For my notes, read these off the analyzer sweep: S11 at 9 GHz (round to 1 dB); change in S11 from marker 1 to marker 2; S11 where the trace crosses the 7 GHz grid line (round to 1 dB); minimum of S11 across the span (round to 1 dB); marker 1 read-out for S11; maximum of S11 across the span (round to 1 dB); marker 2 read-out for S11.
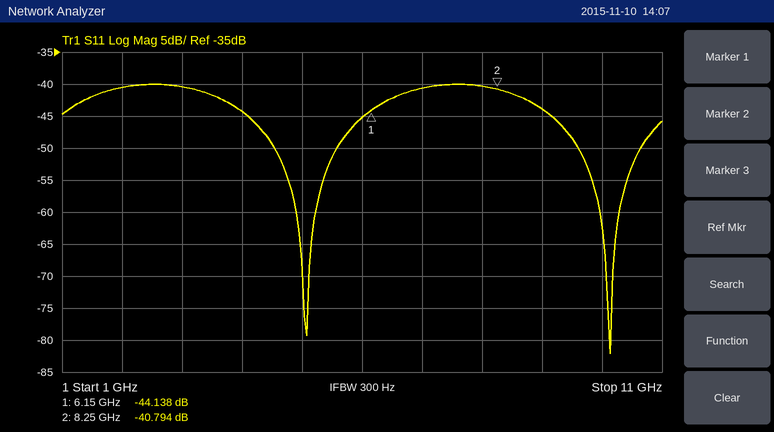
-44 dB
3.344 dB
-41 dB
-82 dB
-44.138 dB
-40 dB
-40.794 dB
